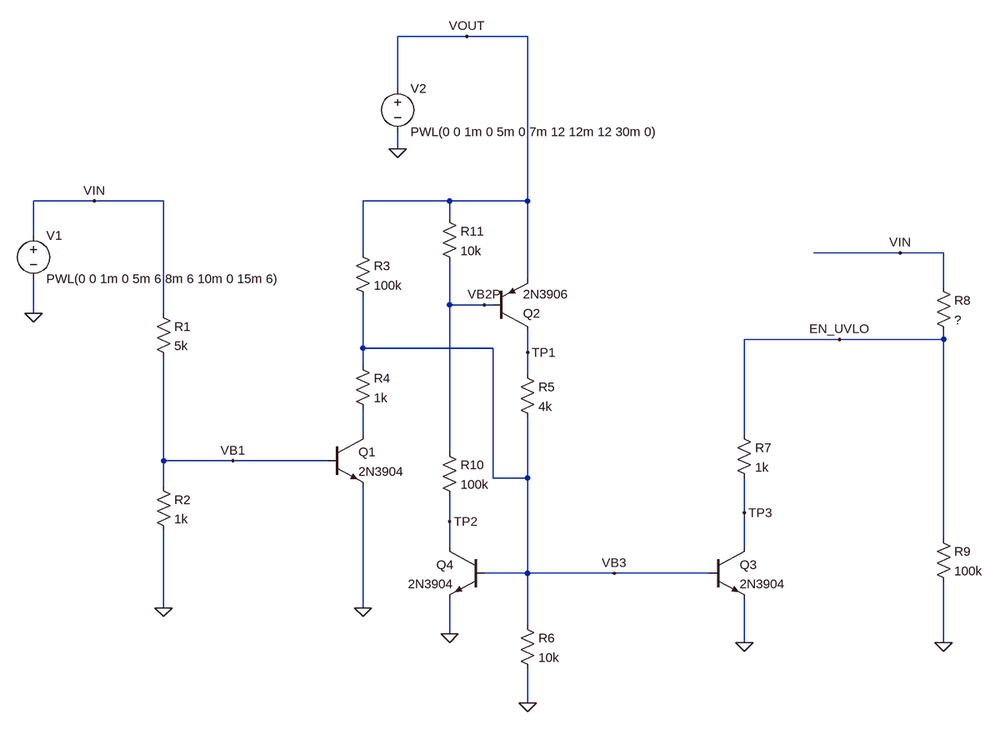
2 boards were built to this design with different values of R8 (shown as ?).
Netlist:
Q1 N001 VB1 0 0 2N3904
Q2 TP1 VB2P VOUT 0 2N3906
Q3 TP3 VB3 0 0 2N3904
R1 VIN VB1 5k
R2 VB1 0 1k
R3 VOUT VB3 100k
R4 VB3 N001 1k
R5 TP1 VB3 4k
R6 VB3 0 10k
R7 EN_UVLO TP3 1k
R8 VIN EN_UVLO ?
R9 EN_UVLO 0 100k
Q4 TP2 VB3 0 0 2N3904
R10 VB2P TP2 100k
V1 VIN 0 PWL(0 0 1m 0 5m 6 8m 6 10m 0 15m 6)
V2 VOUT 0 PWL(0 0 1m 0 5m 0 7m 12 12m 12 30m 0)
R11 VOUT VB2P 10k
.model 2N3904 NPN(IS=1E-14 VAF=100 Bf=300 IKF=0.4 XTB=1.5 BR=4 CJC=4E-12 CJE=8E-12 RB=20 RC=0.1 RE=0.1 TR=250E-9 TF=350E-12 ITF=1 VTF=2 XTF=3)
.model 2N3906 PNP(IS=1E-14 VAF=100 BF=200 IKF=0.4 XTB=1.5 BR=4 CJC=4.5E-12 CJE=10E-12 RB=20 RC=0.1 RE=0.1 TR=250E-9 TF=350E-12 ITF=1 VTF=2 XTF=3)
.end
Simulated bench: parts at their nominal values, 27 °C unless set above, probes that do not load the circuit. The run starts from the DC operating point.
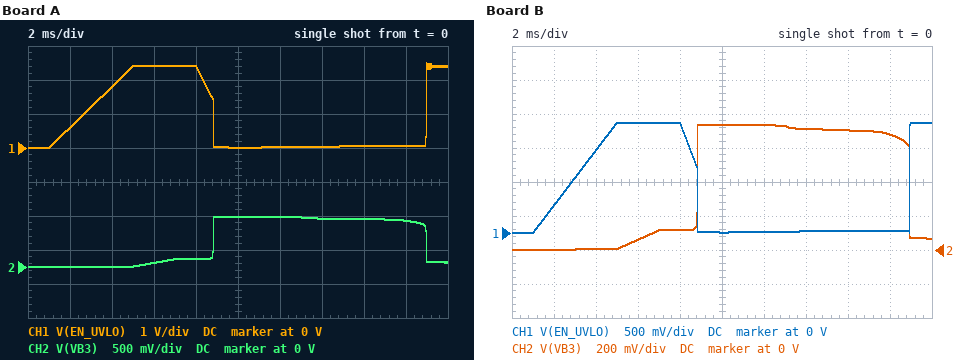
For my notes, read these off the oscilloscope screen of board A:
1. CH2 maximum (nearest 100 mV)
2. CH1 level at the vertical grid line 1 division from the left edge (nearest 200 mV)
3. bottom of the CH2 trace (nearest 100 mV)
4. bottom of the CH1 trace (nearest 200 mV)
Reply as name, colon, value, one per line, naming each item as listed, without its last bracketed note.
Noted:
CH2 maximum: 700 mV
CH1 level at the vertical grid line 1 division from the left edge: 600 mV
bottom of the CH2 trace: 0 V
bottom of the CH1 trace: 0 V
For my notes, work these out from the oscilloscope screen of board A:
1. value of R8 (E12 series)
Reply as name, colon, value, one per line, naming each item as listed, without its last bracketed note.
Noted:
value of R8: 150 kΩ
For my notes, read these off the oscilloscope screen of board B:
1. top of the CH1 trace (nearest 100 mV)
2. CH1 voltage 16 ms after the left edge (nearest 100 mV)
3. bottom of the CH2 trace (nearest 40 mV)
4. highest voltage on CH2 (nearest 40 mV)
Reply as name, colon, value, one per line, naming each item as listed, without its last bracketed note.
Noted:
top of the CH1 trace: 1.6 V
CH1 voltage 16 ms after the left edge: 0 V
bottom of the CH2 trace: 0 V
highest voltage on CH2: 720 mV
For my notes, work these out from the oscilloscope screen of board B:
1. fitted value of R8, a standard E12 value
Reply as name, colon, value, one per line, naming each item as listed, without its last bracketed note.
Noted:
fitted value of R8, a standard E12 value: 270 kΩ
